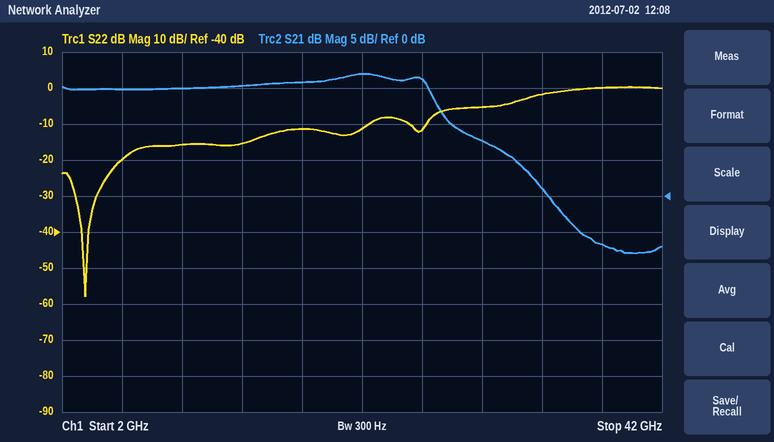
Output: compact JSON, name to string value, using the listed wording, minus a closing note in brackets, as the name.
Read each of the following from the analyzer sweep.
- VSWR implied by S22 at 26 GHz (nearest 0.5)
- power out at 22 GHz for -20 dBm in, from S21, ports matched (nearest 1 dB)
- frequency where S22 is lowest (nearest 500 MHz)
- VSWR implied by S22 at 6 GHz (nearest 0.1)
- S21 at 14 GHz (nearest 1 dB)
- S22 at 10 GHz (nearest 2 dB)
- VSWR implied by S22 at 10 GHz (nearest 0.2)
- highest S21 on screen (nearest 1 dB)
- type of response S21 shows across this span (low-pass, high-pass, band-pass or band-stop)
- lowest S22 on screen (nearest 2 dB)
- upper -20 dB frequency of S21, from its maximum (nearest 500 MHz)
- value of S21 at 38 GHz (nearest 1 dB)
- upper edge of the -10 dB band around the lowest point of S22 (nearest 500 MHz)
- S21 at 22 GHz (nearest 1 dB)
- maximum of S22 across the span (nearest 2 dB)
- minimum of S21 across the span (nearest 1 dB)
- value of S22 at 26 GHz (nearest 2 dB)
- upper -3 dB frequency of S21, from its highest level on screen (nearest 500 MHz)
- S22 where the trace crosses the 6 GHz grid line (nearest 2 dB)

{"VSWR implied by S22 at 26 GHz": "1.5", "power out at 22 GHz for -20 dBm in, from S21, ports matched": "-3 dBm", "frequency where S22 is lowest": "3.5 GHz", "VSWR implied by S22 at 6 GHz": "1.2", "S21 at 14 GHz": "15 dB", "S22 at 10 GHz": "-16 dB", "VSWR implied by S22 at 10 GHz": "1.4", "highest S21 on screen": "17 dB", "type of response S21 shows across this span": "low-pass", "lowest S22 on screen": "-58 dB", "upper -20 dB frequency of S21, from its maximum": "35.5 GHz", "value of S21 at 38 GHz": "-7 dB", "upper edge of the -10 dB band around the lowest point of S22": "22.5 GHz", "S21 at 22 GHz": "17 dB", "maximum of S22 across the span": "0 dB", "minimum of S21 across the span": "-8 dB", "value of S22 at 26 GHz": "-12 dB", "upper -3 dB frequency of S21, from its highest level on screen": "26.5 GHz", "S22 where the trace crosses the 6 GHz grid line": "-20 dB"}
